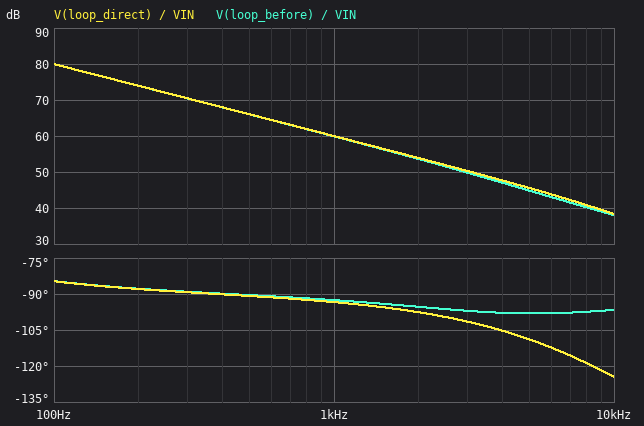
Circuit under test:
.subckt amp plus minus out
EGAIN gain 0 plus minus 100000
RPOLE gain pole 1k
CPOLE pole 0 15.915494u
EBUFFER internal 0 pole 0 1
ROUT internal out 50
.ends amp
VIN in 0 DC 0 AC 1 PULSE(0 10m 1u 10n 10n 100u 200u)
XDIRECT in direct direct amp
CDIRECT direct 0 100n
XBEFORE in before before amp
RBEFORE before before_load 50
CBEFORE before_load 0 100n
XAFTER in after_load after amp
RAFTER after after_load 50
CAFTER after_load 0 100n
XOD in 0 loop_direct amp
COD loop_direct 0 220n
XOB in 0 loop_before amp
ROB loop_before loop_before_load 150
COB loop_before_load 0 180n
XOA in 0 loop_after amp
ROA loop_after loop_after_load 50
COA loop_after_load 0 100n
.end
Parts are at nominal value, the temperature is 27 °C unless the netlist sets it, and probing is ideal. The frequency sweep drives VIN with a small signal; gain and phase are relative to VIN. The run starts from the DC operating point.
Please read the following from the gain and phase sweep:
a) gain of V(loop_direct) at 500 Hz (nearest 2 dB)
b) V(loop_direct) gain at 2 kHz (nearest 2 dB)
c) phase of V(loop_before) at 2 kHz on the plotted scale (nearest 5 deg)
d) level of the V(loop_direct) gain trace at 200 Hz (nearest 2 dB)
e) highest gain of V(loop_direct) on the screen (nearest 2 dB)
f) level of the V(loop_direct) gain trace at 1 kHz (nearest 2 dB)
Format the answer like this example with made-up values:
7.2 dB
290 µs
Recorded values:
66 dB
54 dB
-95 deg
74 dB
80 dB
60 dB
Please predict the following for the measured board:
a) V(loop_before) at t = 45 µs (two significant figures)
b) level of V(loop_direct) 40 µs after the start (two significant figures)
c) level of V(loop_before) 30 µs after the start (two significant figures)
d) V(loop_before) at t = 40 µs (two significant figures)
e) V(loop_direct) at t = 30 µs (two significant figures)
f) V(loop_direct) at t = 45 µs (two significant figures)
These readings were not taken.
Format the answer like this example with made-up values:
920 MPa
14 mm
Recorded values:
2.4 V
1.8 V
1.5 V
2.1 V
1.2 V
2.1 V
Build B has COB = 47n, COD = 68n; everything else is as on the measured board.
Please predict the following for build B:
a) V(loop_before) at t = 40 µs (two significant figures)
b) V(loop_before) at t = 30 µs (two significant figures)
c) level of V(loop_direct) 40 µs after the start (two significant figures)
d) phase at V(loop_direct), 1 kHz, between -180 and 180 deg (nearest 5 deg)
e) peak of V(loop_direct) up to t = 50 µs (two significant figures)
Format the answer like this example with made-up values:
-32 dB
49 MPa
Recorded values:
2.3 V
1.7 V
2.2 V
-90 deg
2.9 V
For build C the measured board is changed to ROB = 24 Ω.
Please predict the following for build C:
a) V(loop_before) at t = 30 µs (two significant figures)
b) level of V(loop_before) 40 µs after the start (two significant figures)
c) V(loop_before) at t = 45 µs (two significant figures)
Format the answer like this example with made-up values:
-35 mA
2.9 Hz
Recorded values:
1.3 V
1.9 V
2.2 V
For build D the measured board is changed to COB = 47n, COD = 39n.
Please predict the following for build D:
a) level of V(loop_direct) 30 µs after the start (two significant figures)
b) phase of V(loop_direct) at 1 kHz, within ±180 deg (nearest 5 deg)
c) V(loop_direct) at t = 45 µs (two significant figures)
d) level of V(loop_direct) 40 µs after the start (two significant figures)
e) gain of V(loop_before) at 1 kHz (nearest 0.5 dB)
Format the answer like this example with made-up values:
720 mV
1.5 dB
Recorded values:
1.7 V
-90 deg
2.6 V
2.3 V
60.0 dB
